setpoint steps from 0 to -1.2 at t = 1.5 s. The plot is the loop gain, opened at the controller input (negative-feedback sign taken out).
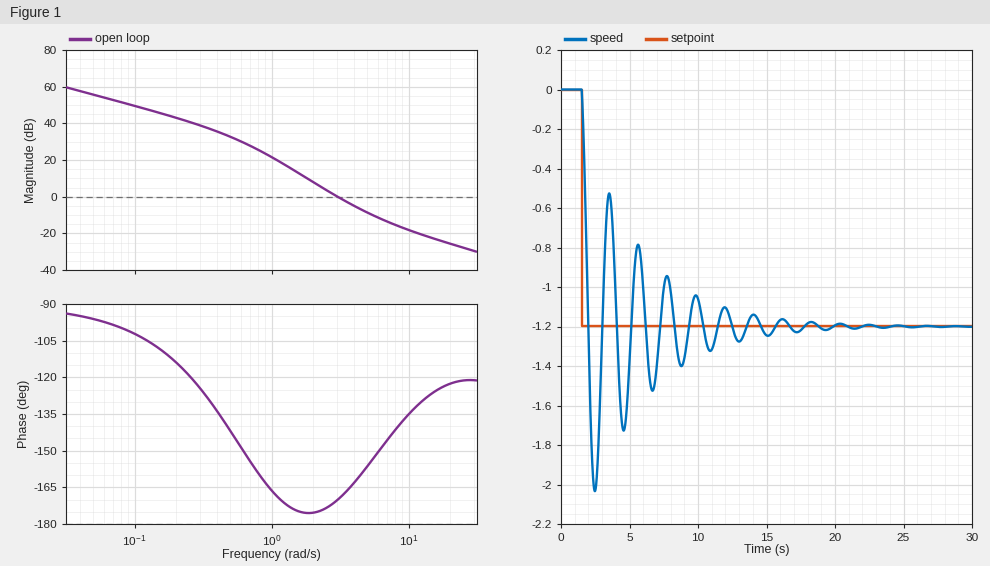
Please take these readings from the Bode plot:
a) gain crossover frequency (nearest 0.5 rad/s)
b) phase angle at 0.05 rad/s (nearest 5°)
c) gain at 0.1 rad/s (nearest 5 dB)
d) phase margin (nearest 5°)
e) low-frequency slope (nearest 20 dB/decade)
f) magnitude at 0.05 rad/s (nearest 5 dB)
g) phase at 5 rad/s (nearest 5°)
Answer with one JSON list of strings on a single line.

["3.0 rad/s", "-95°", "50 dB", "10°", "-20 dB/decade", "55 dB", "-155°"]
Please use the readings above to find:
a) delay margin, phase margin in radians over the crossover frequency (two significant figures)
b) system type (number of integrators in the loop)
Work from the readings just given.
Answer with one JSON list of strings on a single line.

["0.058 s", "1"]
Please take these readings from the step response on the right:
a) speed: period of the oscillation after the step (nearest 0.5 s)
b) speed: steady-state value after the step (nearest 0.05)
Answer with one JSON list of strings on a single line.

["2.0 s", "-1.20"]
